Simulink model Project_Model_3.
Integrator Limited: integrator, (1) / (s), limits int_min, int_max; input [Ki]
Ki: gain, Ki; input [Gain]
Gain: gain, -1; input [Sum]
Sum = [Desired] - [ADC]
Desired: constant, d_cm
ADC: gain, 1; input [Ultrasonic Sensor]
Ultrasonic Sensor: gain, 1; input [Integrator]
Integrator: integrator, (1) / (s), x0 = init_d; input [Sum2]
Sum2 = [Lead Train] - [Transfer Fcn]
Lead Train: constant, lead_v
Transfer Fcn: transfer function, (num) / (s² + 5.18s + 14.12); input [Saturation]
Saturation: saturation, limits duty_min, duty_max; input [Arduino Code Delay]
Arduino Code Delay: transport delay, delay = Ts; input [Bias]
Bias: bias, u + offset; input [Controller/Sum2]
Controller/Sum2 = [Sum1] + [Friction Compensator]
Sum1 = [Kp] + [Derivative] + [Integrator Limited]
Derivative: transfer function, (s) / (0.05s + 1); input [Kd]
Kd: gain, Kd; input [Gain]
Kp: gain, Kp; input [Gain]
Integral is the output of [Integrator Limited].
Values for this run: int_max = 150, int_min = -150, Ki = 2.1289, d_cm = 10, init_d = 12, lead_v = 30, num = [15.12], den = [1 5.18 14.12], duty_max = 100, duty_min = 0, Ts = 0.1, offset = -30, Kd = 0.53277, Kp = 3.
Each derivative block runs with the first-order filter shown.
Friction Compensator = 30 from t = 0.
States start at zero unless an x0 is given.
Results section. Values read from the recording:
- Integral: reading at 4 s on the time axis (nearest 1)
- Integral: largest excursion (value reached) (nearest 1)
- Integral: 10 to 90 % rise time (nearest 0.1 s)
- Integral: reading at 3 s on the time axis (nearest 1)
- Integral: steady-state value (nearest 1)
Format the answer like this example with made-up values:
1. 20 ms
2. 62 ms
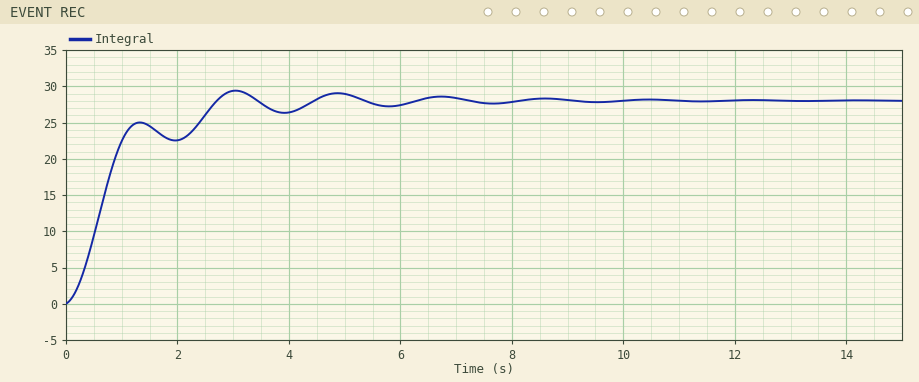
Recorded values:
1. 26
2. 29
3. 2.2 s
4. 29
5. 28
